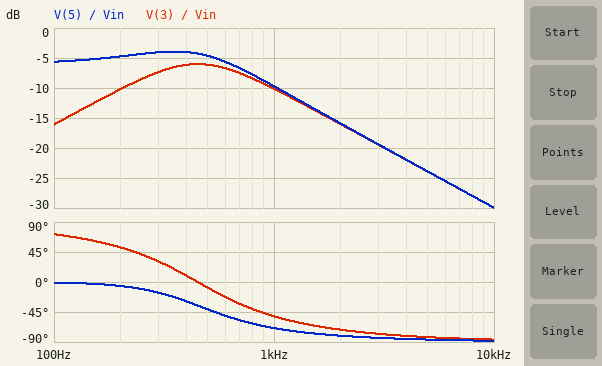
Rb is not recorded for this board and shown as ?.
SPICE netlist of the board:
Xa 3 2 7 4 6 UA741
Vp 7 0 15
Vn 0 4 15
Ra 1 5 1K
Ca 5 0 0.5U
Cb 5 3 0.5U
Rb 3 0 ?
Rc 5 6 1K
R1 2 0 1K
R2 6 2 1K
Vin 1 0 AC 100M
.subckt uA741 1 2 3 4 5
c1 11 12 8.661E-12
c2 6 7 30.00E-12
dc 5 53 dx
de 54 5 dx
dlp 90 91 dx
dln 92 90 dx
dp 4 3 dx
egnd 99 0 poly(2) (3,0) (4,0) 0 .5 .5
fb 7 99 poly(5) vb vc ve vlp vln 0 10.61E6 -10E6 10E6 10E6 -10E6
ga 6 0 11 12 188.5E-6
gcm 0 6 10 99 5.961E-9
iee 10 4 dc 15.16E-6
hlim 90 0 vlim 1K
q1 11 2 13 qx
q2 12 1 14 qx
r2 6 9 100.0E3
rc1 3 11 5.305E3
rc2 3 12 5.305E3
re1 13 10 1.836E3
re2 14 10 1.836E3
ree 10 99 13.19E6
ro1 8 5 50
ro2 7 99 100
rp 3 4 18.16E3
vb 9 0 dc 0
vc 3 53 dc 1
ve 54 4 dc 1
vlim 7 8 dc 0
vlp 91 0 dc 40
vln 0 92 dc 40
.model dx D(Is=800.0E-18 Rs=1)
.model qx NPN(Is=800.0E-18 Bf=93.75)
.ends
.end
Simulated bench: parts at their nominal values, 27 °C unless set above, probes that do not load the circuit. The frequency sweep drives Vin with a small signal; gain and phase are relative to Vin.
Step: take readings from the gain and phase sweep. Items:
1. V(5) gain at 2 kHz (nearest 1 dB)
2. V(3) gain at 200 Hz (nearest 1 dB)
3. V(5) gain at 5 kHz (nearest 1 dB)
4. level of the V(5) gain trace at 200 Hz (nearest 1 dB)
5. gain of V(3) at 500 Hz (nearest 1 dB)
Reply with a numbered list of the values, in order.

1. -16 dB
2. -10 dB
3. -24 dB
4. -5 dB
5. -6 dB
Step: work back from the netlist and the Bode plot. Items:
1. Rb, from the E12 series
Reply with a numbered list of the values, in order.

1. 1 kΩ
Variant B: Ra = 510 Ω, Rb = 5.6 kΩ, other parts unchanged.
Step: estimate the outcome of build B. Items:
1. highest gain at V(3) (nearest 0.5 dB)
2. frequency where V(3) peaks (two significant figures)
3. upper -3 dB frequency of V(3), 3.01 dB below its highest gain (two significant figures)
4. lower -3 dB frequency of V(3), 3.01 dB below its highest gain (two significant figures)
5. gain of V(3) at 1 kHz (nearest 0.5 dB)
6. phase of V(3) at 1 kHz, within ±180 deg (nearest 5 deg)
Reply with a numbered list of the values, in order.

1. 3.5 dB
2. 230 Hz
3. 520 Hz
4. 100 Hz
5. -4.5 dB
6. -65 deg
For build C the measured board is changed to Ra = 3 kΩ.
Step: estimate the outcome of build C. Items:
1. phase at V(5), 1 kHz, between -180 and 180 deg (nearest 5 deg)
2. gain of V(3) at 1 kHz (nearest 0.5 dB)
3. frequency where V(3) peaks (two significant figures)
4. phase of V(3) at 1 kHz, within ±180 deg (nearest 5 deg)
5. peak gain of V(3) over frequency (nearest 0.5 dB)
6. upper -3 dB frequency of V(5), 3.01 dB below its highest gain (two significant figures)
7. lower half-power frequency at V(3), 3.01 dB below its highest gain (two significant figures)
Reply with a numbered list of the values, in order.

1. -80 deg
2. -19.0 dB
3. 370 Hz
4. -65 deg
5. -12.0 dB
6. 530 Hz
7. 210 Hz
